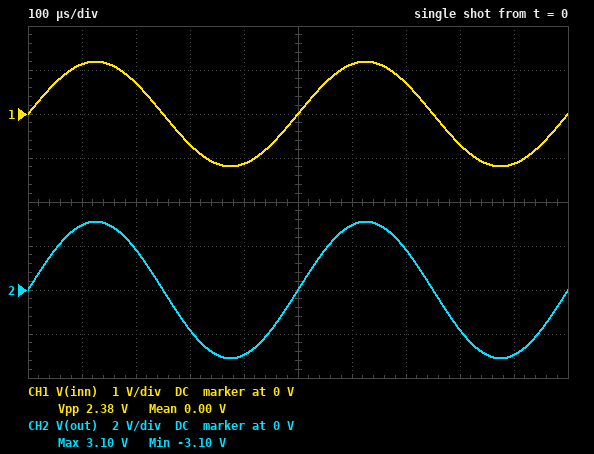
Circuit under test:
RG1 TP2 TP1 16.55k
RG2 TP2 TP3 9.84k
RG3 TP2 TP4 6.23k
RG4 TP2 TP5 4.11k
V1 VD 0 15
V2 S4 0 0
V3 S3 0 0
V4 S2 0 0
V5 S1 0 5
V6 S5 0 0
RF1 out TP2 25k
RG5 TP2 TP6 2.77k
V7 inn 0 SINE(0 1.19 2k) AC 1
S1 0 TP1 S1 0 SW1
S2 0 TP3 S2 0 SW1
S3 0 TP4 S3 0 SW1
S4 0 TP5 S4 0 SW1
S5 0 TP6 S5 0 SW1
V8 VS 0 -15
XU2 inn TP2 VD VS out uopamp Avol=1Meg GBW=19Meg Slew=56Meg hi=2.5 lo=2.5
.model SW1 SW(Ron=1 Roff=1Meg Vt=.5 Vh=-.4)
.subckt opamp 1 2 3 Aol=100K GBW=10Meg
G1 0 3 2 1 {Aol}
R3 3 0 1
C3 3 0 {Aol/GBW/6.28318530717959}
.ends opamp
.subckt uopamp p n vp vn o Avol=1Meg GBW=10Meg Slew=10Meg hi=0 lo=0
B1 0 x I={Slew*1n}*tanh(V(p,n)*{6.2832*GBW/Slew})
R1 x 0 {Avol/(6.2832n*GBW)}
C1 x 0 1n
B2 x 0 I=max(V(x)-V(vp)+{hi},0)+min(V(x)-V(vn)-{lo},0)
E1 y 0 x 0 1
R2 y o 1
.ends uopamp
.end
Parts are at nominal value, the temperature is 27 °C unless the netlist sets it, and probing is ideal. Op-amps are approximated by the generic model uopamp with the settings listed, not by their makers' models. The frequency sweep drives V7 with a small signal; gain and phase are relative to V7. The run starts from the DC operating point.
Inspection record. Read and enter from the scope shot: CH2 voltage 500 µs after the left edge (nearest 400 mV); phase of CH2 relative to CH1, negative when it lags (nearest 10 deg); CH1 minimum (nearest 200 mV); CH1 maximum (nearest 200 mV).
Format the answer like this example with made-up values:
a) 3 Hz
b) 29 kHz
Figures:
a) 0 V
b) 0 deg
c) -1.2 V
d) 1.2 V
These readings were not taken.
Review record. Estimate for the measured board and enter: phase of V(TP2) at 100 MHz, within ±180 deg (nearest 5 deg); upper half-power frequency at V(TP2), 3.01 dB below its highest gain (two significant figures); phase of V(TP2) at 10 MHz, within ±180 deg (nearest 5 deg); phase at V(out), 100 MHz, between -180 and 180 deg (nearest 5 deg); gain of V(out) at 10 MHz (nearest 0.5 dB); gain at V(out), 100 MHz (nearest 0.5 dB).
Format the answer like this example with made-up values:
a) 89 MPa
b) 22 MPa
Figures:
a) -80 deg
b) 17 MHz
c) -30 deg
d) -80 deg
e) -0.5 dB
f) -14.5 dB
